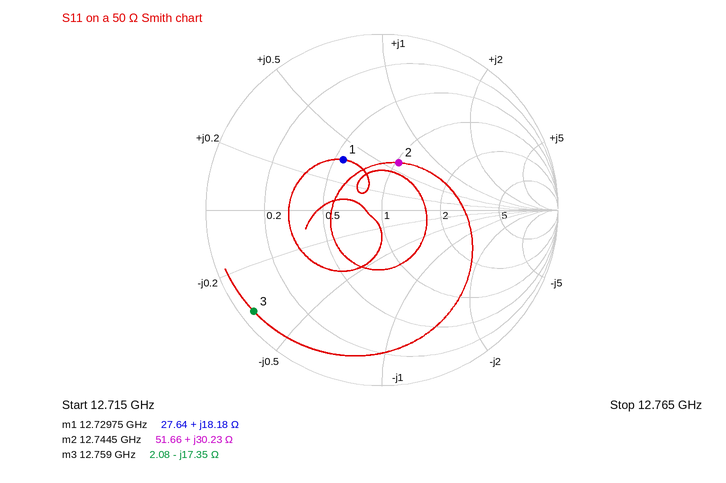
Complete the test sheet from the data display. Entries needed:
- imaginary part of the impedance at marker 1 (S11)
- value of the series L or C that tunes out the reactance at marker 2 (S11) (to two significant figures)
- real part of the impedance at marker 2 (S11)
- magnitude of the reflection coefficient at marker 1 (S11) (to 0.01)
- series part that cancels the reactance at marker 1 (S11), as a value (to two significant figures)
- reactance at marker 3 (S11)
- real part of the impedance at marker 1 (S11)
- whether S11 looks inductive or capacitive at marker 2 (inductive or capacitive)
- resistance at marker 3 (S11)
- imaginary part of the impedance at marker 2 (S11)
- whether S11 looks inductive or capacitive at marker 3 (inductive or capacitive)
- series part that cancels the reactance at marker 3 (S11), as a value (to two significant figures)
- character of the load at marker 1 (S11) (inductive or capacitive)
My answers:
+18.18 Ω
410 fF
51.66 Ω
0.36
690 fF
-17.35 Ω
27.64 Ω
inductive
2.08 Ω
+30.23 Ω
capacitive
220 pH
inductive
